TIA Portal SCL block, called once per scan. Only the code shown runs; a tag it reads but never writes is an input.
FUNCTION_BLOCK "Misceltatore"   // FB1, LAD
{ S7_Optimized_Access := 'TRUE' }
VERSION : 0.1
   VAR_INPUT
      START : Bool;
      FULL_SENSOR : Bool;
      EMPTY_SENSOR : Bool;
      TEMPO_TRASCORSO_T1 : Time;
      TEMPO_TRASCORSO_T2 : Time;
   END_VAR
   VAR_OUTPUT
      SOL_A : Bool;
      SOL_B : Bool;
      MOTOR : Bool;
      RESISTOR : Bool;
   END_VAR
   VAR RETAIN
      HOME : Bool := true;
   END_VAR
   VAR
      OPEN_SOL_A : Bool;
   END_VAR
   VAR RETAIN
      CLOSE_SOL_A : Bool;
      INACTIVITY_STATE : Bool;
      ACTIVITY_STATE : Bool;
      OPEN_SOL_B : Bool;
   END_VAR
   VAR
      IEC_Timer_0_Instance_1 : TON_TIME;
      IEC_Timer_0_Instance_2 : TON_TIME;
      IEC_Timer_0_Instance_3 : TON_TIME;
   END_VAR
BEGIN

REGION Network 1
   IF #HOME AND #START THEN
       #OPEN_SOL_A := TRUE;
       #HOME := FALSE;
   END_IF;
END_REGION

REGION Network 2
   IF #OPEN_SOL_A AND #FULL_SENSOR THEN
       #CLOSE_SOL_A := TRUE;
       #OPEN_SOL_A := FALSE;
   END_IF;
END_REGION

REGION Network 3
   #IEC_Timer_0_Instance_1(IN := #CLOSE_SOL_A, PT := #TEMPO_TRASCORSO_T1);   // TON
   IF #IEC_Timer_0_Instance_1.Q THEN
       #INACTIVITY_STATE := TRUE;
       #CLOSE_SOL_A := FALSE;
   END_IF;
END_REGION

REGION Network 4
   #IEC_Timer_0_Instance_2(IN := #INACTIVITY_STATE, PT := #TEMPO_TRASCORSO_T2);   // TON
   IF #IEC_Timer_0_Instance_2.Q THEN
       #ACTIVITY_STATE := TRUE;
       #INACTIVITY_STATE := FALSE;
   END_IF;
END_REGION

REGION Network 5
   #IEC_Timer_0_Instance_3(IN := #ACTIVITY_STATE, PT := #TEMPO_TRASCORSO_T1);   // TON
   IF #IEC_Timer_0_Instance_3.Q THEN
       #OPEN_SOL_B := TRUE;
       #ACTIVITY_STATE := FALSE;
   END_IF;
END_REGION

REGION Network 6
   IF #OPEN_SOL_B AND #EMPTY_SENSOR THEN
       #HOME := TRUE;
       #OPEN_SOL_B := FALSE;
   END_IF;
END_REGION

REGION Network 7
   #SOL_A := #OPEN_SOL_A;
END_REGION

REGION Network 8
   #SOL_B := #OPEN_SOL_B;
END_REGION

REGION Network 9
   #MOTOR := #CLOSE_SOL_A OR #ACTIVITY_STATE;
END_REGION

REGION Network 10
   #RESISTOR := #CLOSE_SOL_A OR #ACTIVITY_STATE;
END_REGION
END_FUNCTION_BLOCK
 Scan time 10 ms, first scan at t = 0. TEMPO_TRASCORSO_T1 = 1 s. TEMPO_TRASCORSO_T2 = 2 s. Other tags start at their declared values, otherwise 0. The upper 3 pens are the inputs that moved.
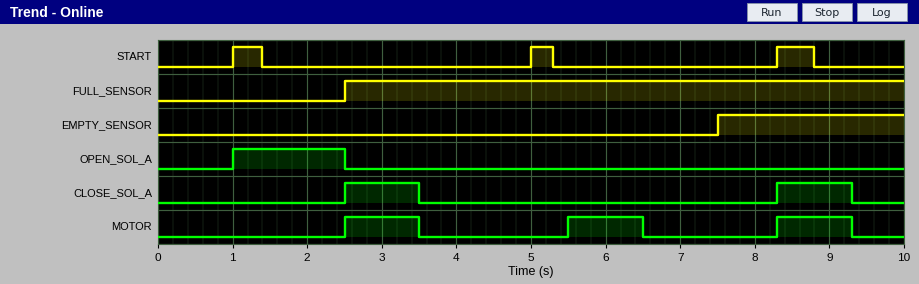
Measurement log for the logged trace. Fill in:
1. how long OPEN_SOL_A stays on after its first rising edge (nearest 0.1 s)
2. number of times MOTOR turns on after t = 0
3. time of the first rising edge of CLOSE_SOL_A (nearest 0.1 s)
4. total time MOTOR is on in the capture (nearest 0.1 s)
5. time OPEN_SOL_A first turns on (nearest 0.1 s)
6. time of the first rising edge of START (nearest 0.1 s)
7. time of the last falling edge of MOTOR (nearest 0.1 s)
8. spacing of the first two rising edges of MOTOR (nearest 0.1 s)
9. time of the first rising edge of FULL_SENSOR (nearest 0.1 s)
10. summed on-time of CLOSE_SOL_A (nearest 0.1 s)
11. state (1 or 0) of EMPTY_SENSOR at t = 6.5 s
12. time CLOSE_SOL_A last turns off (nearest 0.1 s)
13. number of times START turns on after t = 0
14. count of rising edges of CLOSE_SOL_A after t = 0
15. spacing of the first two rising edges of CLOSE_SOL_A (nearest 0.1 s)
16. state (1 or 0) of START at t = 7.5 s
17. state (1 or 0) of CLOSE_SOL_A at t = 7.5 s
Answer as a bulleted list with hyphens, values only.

- 1.5 s
- 3
- 2.5 s
- 3.0 s
- 1.0 s
- 1.0 s
- 9.3 s
- 3.0 s
- 2.5 s
- 2.0 s
- 0
- 9.3 s
- 3
- 2
- 5.8 s
- 0
- 0
